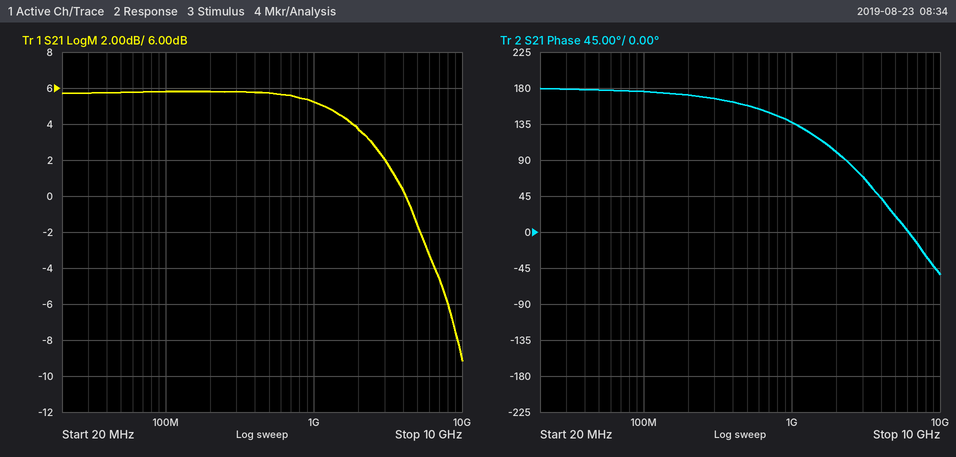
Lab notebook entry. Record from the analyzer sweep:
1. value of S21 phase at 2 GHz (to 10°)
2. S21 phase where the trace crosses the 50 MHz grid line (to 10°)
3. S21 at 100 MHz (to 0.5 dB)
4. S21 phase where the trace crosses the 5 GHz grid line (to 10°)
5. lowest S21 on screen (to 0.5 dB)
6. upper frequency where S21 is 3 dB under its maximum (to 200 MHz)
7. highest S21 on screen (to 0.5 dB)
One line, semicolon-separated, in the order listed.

100°; 180°; 6.0 dB; 20°; -9.0 dB; 2.6 GHz; 6.0 dB
